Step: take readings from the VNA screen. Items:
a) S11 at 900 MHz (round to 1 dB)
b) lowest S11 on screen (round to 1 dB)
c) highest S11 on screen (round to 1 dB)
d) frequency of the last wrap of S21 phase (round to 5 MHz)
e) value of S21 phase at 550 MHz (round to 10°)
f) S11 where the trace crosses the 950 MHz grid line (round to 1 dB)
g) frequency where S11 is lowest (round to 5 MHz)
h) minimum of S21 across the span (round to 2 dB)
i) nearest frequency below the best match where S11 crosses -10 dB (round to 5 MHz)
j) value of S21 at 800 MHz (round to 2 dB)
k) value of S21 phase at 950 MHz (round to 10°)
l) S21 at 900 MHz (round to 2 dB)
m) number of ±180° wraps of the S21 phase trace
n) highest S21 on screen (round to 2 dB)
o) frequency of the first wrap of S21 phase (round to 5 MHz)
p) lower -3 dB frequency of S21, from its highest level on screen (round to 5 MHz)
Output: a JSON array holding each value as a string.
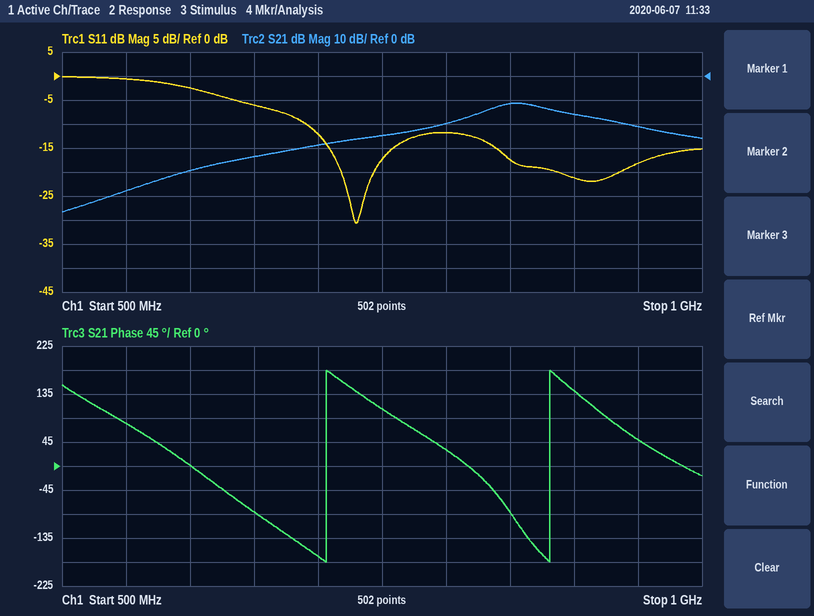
["-21 dB", "-31 dB", "0 dB", "880 MHz", "80°", "-18 dB", "730 MHz", "-56 dB", "690 MHz", "-20 dB", "50°", "-16 dB", "2", "-12 dB", "705 MHz", "830 MHz"]
